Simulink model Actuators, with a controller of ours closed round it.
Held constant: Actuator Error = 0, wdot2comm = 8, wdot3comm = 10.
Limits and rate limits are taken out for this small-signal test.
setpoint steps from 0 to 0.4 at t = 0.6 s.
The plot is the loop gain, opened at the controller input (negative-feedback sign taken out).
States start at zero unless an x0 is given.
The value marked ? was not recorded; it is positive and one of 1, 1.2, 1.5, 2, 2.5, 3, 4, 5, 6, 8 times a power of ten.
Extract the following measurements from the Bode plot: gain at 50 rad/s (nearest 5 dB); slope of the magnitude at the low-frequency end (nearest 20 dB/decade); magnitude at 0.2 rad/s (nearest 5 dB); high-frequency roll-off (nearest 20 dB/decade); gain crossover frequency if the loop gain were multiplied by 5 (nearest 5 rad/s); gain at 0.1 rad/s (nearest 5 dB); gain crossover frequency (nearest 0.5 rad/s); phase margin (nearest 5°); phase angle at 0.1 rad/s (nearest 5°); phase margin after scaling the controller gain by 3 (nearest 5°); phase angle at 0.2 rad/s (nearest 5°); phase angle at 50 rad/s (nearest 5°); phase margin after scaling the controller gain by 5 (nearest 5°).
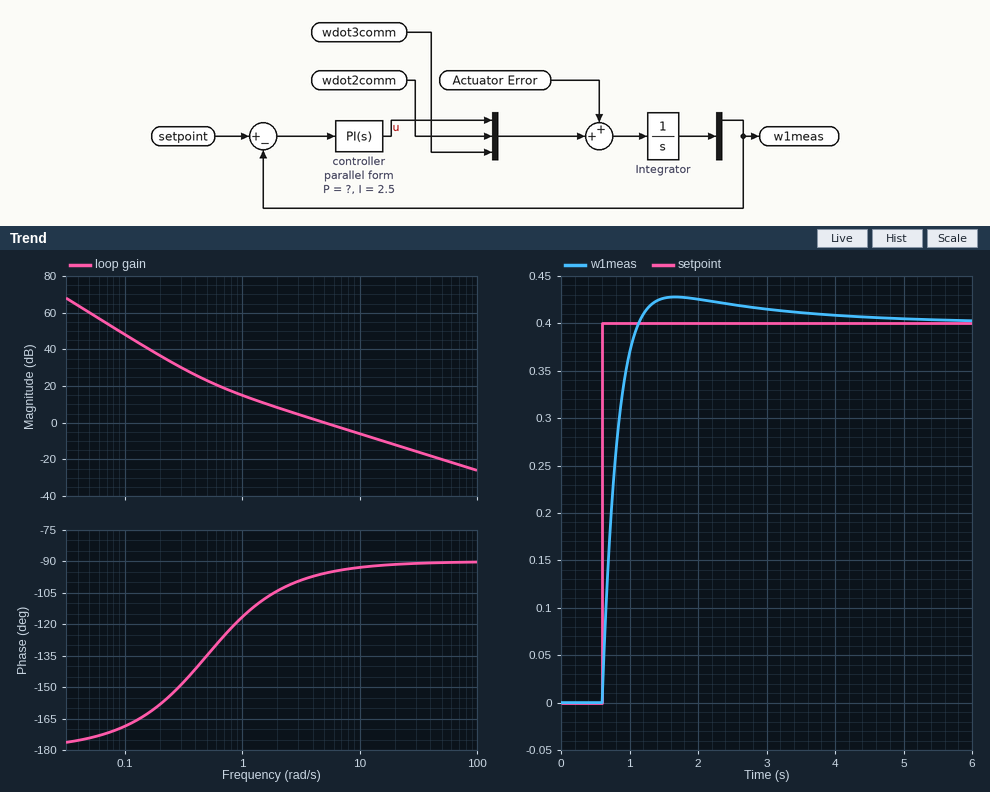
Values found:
-20 dB
-40 dB/decade
35 dB
-20 dB/decade
25 rad/s
50 dB
5.0 rad/s
85°
-170°
90°
-160°
-90°
90°
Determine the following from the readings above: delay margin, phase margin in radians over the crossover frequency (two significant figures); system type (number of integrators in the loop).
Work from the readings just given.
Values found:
0.30 s
2
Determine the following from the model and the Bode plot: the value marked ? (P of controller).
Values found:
5
